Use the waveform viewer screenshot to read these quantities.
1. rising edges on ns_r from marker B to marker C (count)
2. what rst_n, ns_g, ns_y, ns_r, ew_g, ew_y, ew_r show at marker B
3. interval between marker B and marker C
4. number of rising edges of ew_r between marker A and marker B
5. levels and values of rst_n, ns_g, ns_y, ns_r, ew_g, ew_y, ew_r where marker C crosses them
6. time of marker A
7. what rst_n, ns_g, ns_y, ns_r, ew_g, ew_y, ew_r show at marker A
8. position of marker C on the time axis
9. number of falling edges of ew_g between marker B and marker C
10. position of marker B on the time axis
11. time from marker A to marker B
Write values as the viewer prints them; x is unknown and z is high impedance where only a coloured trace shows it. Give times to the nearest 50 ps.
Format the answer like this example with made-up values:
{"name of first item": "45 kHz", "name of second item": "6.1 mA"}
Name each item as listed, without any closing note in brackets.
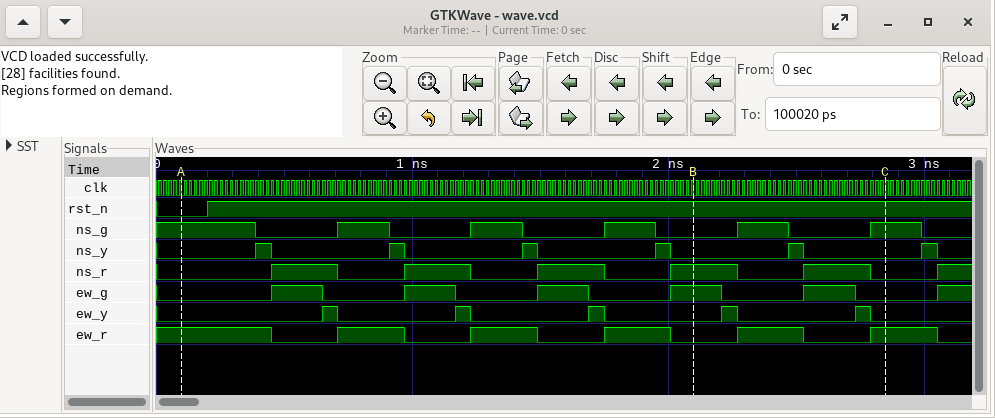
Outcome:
{"rising edges on ns_r from marker B to marker C": "1", "what rst_n, ns_g, ns_y, ns_r, ew_g, ew_y, ew_r show at marker B": "rst_n=1, ns_g=0, ns_y=0, ns_r=1, ew_g=1, ew_y=0, ew_r=0", "interval between marker B and marker C": "750 ps", "number of rising edges of ew_r between marker A and marker B": "3", "levels and values of rst_n, ns_g, ns_y, ns_r, ew_g, ew_y, ew_r where marker C crosses them": "rst_n=1, ns_g=1, ns_y=0, ns_r=0, ew_g=0, ew_y=0, ew_r=1", "time of marker A": "100 ps", "what rst_n, ns_g, ns_y, ns_r, ew_g, ew_y, ew_r show at marker A": "rst_n=0, ns_g=1, ns_y=0, ns_r=0, ew_g=0, ew_y=0, ew_r=1", "position of marker C on the time axis": "2850 ps", "number of falling edges of ew_g between marker B and marker C": "2", "position of marker B on the time axis": "2100 ps", "time from marker A to marker B": "2000 ps"}
